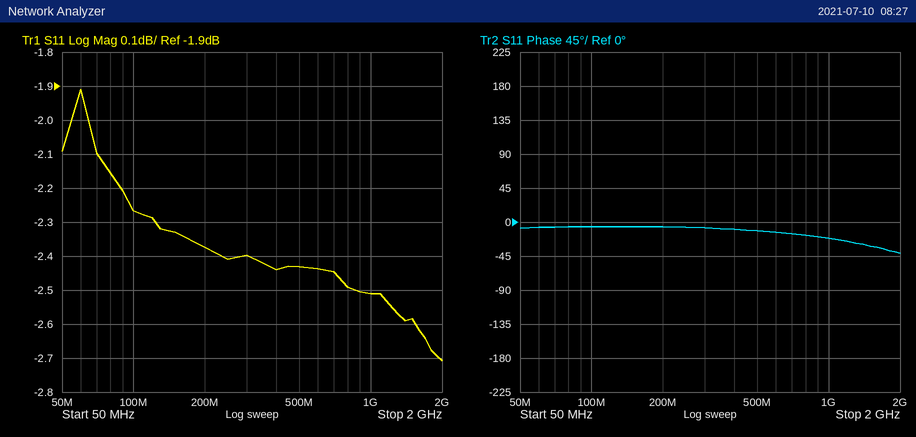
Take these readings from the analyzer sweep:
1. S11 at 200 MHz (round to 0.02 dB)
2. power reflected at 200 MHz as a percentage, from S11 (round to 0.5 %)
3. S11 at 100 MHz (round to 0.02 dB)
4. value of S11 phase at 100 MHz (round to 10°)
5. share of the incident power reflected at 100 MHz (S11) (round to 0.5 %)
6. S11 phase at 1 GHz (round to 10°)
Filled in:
-2.38 dB
58.0 %
-2.26 dB
-10°
59.5 %
-20°
